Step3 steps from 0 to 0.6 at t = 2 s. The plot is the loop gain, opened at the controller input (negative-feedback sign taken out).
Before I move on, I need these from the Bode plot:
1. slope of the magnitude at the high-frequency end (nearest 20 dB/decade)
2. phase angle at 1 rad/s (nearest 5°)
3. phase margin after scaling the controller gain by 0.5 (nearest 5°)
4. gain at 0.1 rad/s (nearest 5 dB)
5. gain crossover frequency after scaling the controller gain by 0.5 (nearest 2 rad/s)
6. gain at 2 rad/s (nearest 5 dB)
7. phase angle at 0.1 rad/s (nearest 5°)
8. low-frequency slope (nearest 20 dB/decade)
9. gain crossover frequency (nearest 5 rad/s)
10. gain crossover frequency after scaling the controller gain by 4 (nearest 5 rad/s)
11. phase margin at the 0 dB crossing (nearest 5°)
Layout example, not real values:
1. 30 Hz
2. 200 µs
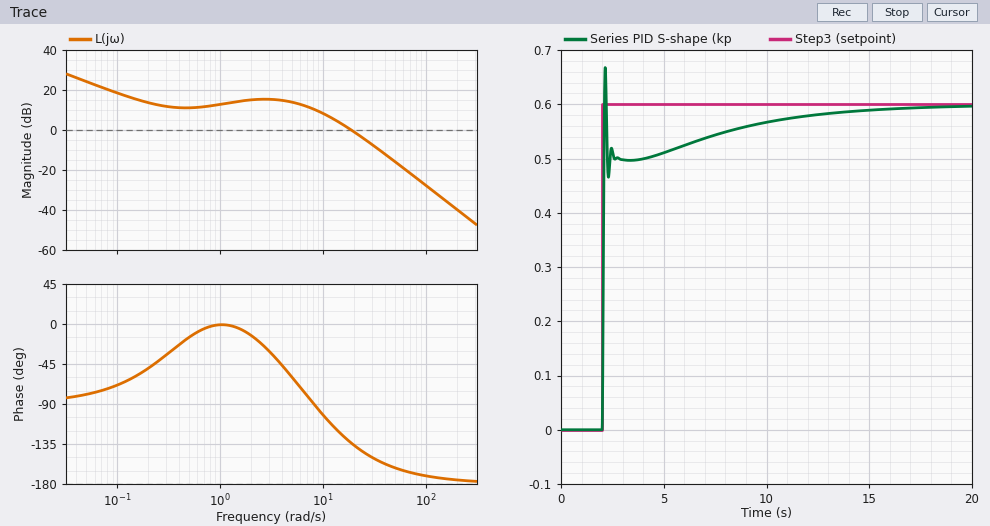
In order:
1. -40 dB/decade
2. 0°
3. 65°
4. 20 dB
5. 12 rad/s
6. 15 dB
7. -70°
8. -20 dB/decade
9. 20 rad/s
10. 40 rad/s
11. 45°
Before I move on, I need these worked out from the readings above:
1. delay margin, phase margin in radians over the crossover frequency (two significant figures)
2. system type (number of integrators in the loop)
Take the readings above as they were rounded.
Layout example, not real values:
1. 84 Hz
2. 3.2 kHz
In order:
1. 0.039 s
2. 1
